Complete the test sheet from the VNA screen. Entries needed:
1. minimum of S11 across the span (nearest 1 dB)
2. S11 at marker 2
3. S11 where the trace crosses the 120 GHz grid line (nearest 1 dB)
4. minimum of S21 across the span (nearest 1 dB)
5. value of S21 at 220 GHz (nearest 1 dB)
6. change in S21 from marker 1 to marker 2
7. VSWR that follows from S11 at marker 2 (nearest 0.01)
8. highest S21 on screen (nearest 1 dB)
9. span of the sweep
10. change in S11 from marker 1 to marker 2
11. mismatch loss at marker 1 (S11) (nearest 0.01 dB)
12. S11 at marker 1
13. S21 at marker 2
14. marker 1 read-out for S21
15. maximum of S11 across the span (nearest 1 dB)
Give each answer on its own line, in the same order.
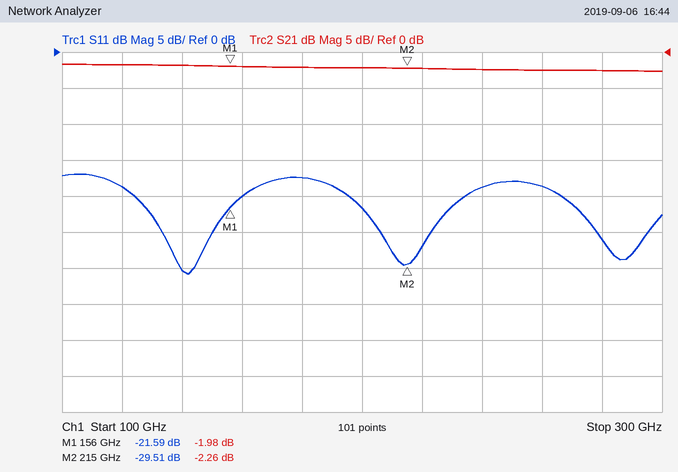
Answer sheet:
-31 dB
-29.51 dB
-19 dB
-3 dB
-2 dB
-0.28 dB
1.07
-2 dB
200 GHz
-7.92 dB
0.03 dB
-21.59 dB
-2.26 dB
-1.98 dB
-17 dB
